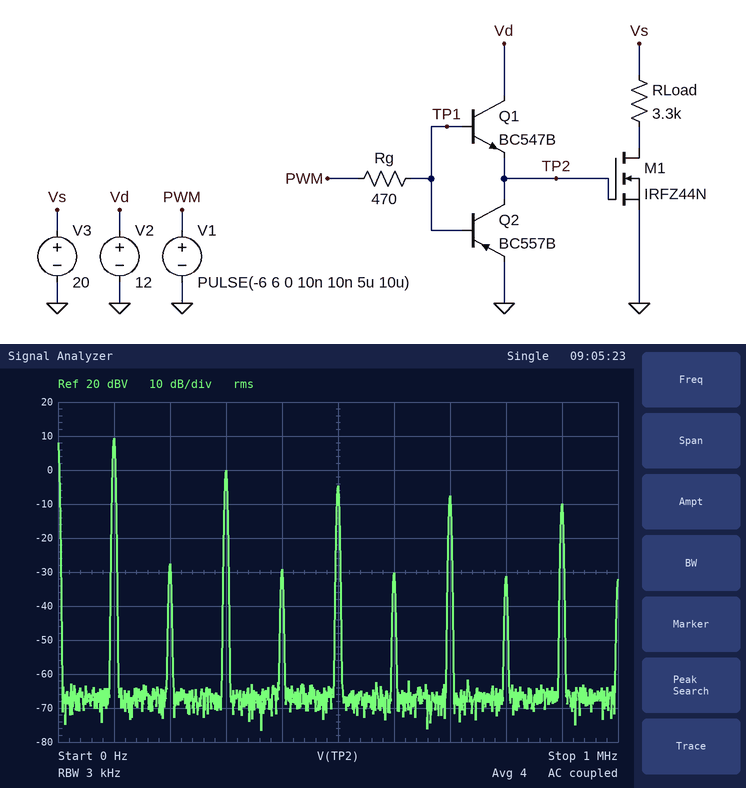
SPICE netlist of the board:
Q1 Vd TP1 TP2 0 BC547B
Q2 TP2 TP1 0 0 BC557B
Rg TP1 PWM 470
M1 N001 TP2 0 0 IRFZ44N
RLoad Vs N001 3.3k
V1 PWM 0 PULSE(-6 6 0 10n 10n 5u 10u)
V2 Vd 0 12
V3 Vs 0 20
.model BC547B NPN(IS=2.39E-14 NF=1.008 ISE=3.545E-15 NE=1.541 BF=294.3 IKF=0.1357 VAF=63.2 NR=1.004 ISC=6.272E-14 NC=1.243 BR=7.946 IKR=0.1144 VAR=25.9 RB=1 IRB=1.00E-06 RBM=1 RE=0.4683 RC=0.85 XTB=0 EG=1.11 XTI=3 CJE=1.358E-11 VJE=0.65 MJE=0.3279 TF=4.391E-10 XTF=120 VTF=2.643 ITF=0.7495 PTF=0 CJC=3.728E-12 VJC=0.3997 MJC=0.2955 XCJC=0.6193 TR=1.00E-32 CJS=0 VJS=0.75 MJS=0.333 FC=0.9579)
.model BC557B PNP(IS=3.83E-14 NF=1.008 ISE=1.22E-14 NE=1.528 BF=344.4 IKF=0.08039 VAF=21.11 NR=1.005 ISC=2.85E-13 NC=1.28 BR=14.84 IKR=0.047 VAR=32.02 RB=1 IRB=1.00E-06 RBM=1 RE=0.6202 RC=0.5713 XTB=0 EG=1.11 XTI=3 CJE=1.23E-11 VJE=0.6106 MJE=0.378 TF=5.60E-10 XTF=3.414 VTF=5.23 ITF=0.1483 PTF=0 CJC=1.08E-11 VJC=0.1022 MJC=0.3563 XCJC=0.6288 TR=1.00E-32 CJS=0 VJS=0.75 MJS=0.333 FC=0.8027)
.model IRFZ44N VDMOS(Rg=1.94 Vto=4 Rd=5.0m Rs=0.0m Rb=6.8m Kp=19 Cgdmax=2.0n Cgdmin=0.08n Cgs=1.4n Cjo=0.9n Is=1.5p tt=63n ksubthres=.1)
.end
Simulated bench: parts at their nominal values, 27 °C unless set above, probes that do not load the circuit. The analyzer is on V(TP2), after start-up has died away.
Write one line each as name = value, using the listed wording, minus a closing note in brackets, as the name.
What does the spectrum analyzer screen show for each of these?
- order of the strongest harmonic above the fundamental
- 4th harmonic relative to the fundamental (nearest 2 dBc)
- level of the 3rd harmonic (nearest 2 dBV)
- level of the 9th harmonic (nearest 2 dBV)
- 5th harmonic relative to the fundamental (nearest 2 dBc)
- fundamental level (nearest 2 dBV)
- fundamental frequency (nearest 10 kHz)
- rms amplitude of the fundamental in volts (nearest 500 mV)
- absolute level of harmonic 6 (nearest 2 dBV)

order of the strongest harmonic above the fundamental = 3
4th harmonic relative to the fundamental = -38 dBc
level of the 3rd harmonic = 0 dBV
level of the 9th harmonic = -10 dBV
5th harmonic relative to the fundamental = -14 dBc
fundamental level = 10 dBV
fundamental frequency = 100 kHz
rms amplitude of the fundamental in volts = 3.0 V
absolute level of harmonic 6 = -30 dBV
